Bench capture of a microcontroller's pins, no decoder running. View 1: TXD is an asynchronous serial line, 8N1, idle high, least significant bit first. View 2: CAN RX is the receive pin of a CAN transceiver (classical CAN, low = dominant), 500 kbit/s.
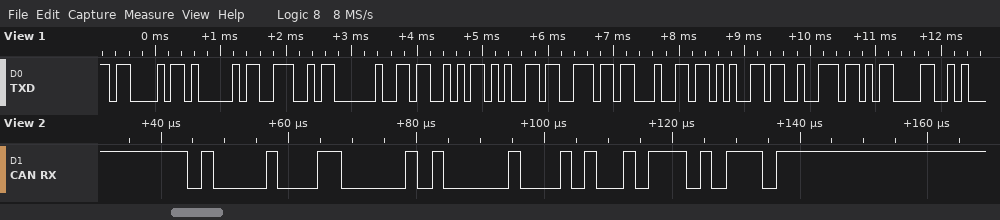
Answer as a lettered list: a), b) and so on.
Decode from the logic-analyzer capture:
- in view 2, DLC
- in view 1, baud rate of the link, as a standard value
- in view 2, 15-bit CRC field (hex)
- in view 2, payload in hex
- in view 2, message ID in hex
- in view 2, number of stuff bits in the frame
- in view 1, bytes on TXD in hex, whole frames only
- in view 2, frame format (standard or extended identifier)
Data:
a) 1
b) 9600 baud
c) 0x52EB
d) 00
e) 0x423
f) 2
g) 0x43 0x41 0x4E 0x20 0x53 0x65 0x6E 0x64 0x65 0x72 0x0D
h) standard
